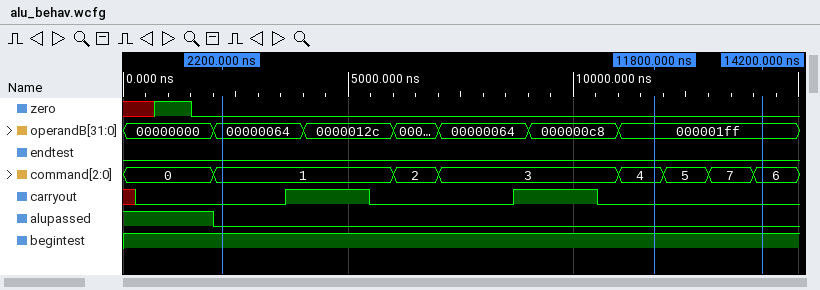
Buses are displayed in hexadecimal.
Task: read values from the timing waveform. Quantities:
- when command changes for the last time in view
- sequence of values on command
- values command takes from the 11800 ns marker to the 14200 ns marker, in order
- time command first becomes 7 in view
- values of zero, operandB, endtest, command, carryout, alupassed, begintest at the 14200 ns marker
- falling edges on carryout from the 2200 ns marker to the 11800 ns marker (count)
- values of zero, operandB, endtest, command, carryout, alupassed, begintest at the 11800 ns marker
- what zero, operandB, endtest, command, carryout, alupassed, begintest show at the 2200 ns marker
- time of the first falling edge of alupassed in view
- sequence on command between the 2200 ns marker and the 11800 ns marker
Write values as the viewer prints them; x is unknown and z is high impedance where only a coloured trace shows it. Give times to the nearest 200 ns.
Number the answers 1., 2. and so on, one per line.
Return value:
1. 14000 ns
2. 0, 1, 2, 3, 4, 5, 7, 6
3. 4, 5, 7, 6
4. 13000 ns
5. zero=0, operandB=000001ff, endtest=0, command=6, carryout=0, alupassed=0, begintest=1
6. 2
7. zero=0, operandB=000001ff, endtest=0, command=4, carryout=0, alupassed=0, begintest=1
8. zero=0, operandB=00000064, endtest=0, command=1, carryout=0, alupassed=0, begintest=1
9. 2000 ns
10. 1, 2, 3, 4
